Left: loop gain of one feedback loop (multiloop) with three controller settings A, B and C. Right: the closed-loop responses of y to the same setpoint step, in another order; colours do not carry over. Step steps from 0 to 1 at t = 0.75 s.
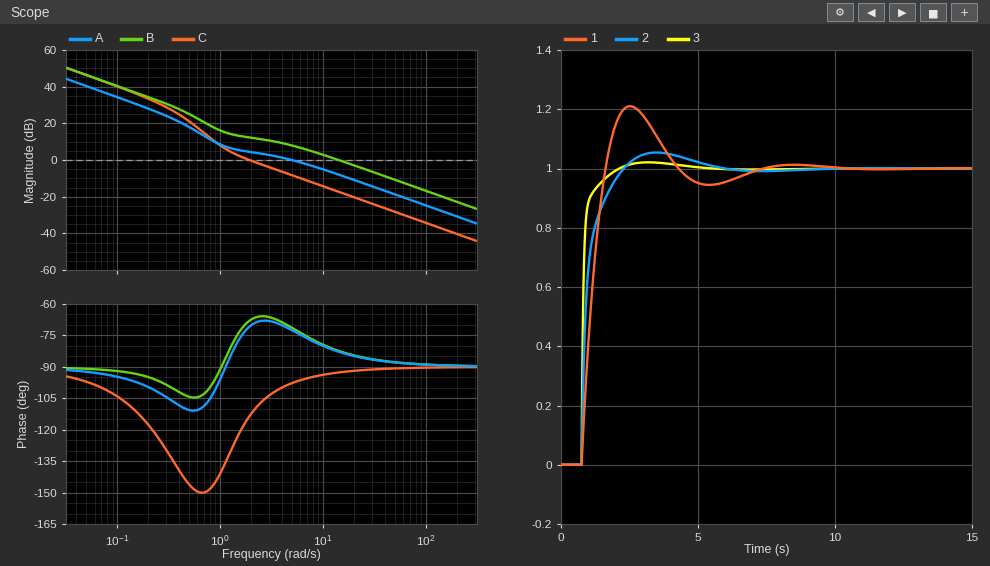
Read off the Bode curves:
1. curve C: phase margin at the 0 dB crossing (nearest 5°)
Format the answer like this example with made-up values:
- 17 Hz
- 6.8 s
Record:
- 65°
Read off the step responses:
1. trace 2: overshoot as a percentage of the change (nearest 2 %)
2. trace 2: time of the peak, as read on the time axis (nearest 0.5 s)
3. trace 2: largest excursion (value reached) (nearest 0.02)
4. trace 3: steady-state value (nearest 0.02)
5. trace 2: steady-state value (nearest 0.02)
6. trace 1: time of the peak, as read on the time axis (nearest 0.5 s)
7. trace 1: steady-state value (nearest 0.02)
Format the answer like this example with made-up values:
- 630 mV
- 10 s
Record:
- 6 %
- 3.5 s
- 1.06
- 1.00
- 1.00
- 2.5 s
- 1.00
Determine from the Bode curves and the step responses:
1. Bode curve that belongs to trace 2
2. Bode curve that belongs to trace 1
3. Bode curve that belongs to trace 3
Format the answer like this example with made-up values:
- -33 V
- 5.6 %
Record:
- A
- C
- B
